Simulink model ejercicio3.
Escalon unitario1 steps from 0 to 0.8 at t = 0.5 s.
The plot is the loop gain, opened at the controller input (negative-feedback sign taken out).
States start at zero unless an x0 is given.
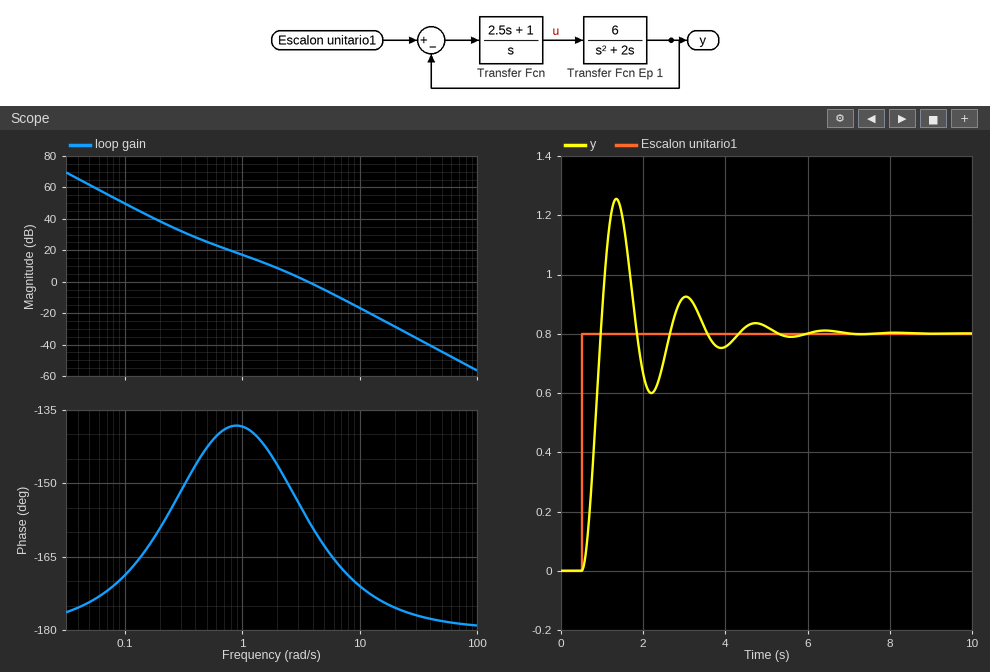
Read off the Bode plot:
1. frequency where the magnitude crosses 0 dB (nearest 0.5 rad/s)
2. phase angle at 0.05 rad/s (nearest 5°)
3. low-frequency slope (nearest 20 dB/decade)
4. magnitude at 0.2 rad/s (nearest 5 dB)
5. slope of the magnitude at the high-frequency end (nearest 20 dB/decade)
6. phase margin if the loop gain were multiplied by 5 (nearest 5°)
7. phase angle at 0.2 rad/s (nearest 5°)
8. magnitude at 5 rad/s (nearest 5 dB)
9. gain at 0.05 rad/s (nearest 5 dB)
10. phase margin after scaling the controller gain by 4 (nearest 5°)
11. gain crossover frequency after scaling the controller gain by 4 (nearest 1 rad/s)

3.5 rad/s
-175°
-40 dB/decade
40 dB
-40 dB/decade
10°
-160°
-5 dB
60 dB
10°
8 rad/s
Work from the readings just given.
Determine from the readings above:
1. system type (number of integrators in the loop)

2
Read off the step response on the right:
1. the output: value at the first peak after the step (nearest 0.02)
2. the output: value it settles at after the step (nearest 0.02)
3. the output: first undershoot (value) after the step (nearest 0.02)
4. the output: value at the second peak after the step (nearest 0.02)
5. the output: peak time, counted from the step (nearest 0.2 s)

1.26
0.80
0.60
0.92
0.8 s
